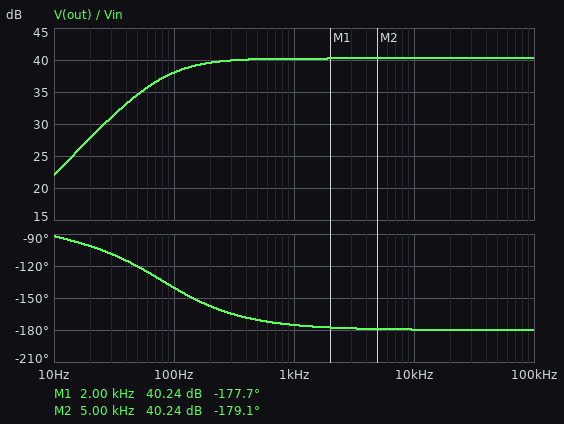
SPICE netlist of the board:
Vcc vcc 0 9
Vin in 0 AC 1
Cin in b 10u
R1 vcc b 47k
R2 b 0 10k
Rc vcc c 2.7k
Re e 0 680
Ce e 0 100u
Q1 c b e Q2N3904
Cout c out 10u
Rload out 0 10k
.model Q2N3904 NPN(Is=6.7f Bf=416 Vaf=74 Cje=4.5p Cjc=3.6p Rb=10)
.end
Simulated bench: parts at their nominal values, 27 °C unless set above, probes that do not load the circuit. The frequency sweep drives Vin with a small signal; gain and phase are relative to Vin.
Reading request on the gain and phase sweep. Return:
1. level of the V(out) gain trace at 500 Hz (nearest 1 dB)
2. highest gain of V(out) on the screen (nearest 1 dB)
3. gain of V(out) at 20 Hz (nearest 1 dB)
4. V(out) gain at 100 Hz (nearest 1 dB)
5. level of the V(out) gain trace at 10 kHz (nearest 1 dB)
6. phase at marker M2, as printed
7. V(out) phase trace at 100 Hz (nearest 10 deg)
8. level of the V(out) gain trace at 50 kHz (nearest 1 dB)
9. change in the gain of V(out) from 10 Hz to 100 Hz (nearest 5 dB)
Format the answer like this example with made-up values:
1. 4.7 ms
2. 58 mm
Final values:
1. 40 dB
2. 40 dB
3. 28 dB
4. 38 dB
5. 40 dB
6. -179.1 deg
7. -140 deg
8. 40 dB
9. 15 dB
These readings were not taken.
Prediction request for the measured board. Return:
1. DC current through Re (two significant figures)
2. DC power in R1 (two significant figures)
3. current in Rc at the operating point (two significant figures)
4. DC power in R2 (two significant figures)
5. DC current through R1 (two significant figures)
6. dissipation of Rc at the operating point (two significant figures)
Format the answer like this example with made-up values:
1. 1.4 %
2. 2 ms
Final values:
1. 1.3 mA
2. 1.2 mW
3. 1.3 mA
4. 240 µW
5. 160 µA
6. 4.5 mW
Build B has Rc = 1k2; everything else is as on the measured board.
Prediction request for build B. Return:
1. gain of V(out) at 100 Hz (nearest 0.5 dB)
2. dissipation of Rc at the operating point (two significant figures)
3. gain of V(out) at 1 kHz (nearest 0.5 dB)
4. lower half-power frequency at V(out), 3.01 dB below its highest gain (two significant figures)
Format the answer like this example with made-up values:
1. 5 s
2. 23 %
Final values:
1. 32.0 dB
2. 2.0 mW
3. 34.5 dB
4. 83 Hz
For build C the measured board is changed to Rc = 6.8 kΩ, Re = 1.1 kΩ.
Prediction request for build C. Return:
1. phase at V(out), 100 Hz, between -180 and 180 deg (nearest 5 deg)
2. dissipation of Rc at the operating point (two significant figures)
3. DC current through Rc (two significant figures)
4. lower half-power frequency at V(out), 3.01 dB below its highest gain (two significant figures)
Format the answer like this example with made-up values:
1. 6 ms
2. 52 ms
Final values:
1. -150 deg
2. 4.6 mW
3. 820 µA
4. 51 Hz
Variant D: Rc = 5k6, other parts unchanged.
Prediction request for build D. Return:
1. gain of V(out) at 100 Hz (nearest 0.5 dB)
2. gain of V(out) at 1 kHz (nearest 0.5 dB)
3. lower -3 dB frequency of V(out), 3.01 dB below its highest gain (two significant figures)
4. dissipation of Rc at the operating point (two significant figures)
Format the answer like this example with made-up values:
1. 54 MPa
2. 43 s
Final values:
1. 42.5 dB
2. 44.5 dB
3. 79 Hz
4. 9.4 mW
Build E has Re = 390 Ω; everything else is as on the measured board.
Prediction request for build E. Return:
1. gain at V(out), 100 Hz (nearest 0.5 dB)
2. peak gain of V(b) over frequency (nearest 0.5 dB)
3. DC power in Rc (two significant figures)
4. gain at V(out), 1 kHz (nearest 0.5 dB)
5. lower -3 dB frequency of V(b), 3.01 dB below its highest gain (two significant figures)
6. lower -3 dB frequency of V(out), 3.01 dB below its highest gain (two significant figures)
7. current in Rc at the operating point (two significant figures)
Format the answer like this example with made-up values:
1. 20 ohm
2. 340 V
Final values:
1. 40.0 dB
2. 0 dB
3. 13 mW
4. 44.5 dB
5. 2.1 Hz
6. 130 Hz
7. 2.2 mA
